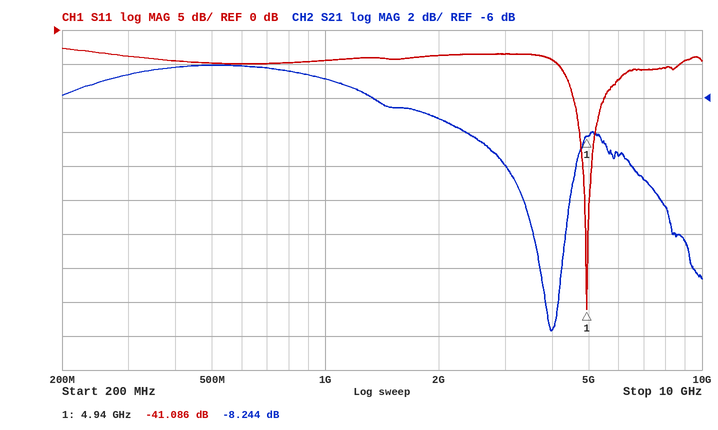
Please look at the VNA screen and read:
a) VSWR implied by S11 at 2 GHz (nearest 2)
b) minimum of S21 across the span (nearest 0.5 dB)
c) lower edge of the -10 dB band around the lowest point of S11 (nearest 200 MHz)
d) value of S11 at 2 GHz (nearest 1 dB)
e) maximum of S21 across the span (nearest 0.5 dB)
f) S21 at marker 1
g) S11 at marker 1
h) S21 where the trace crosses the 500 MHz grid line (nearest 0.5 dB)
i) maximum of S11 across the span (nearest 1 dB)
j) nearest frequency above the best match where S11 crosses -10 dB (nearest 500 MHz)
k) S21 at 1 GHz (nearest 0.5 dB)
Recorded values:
4
-19.5 dB
4.6 GHz
-4 dB
-4.0 dB
-8.244 dB
-41.086 dB
-4.0 dB
-3 dB
5.5 GHz
-5.0 dB
